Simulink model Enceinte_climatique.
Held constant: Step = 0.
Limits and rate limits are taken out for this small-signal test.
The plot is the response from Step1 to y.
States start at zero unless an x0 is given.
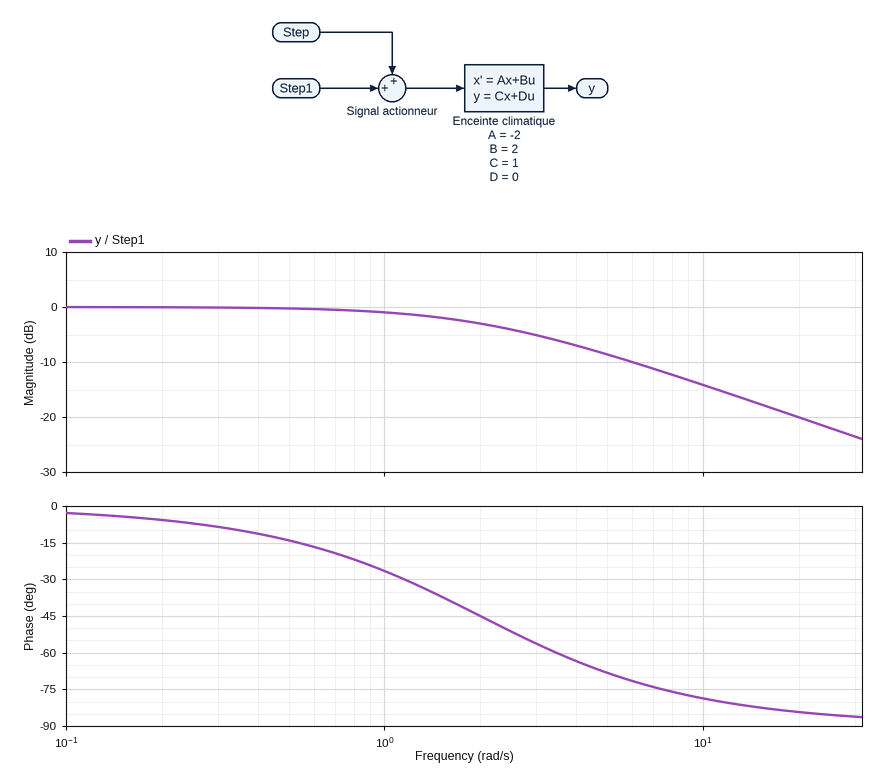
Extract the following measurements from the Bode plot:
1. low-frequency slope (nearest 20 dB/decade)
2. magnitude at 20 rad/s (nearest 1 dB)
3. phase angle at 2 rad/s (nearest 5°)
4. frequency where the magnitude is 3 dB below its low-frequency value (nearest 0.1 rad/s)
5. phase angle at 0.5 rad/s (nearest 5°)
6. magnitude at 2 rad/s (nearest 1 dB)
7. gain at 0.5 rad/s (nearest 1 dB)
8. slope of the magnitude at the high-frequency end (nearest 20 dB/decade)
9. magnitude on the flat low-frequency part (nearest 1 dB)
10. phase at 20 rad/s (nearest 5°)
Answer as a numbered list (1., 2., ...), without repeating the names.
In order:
1. 0 dB/decade
2. -20 dB
3. -45°
4. 2.0 rad/s
5. -15°
6. -3 dB
7. 0 dB
8. -20 dB/decade
9. 0 dB
10. -85°
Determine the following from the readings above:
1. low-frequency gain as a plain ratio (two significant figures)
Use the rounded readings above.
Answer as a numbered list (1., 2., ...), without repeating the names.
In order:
1. 1.0
